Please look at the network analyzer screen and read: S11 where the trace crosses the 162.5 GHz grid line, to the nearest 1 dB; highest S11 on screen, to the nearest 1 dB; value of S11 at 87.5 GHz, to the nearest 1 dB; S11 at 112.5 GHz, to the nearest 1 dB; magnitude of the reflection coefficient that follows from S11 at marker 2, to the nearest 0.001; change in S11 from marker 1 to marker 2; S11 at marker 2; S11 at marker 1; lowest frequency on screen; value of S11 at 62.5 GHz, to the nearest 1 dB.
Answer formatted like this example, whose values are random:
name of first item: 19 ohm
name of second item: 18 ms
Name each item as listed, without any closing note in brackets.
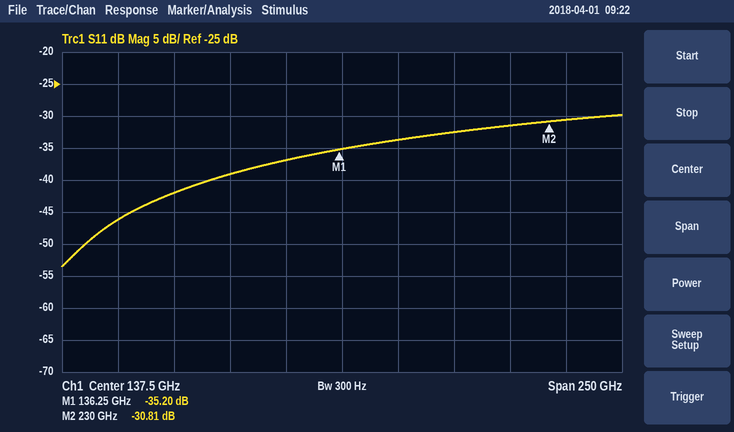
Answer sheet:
S11 where the trace crosses the 162.5 GHz grid line, to the nearest 1 dB: -34 dB
highest S11 on screen, to the nearest 1 dB: -30 dB
value of S11 at 87.5 GHz, to the nearest 1 dB: -39 dB
S11 at 112.5 GHz, to the nearest 1 dB: -37 dB
magnitude of the reflection coefficient that follows from S11 at marker 2, to the nearest 0.001: 0.029
change in S11 from marker 1 to marker 2: 4.39 dB
S11 at marker 2: -30.81 dB
S11 at marker 1: -35.20 dB
lowest frequency on screen: 12.5 GHz
value of S11 at 62.5 GHz, to the nearest 1 dB: -42 dB
